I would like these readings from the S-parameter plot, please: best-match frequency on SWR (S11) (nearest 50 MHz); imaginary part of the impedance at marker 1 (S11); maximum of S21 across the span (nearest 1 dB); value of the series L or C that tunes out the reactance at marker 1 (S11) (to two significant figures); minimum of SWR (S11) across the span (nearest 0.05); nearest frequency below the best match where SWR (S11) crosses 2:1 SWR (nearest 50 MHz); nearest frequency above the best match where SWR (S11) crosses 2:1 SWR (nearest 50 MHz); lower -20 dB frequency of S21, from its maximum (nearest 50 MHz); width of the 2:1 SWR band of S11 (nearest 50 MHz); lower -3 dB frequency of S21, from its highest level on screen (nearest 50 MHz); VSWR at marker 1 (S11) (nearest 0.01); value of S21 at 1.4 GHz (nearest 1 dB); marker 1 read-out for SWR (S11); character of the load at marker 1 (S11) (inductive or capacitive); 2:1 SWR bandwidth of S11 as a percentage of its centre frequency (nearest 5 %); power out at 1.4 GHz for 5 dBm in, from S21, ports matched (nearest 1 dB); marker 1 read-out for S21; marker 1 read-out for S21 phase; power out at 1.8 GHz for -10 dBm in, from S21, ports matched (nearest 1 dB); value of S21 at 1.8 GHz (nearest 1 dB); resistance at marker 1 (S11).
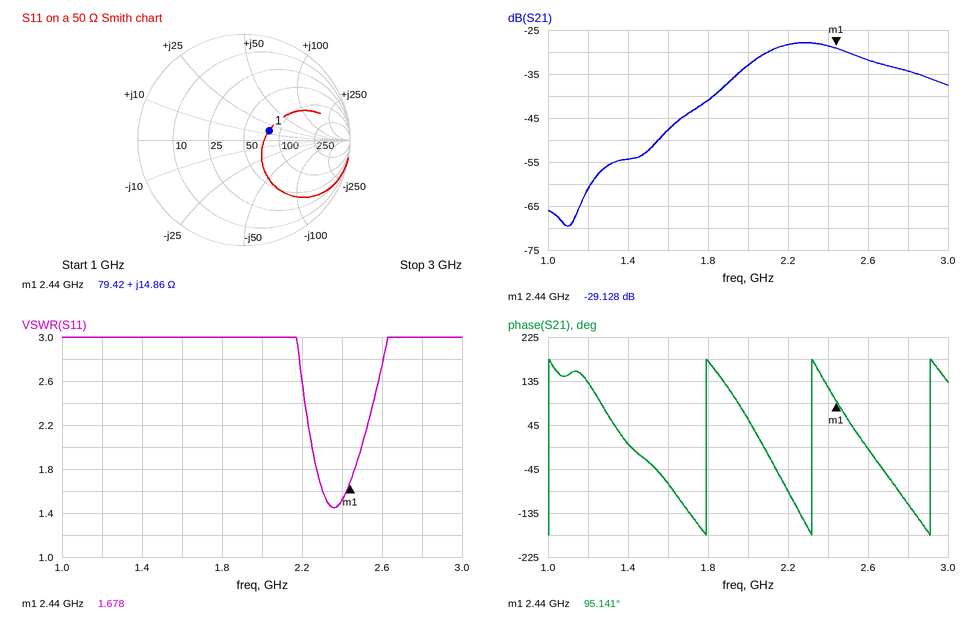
2.35 GHz
+14.86 Ω
-28 dB
4.4 pF
1.45
2.25 GHz
2.50 GHz
1.60 GHz
250 MHz
2.05 GHz
1.68
-54 dB
1.678
inductive
10 %
-49 dBm
-29.128 dB
95.141°
-51 dBm
-41 dB
79.42 Ω
